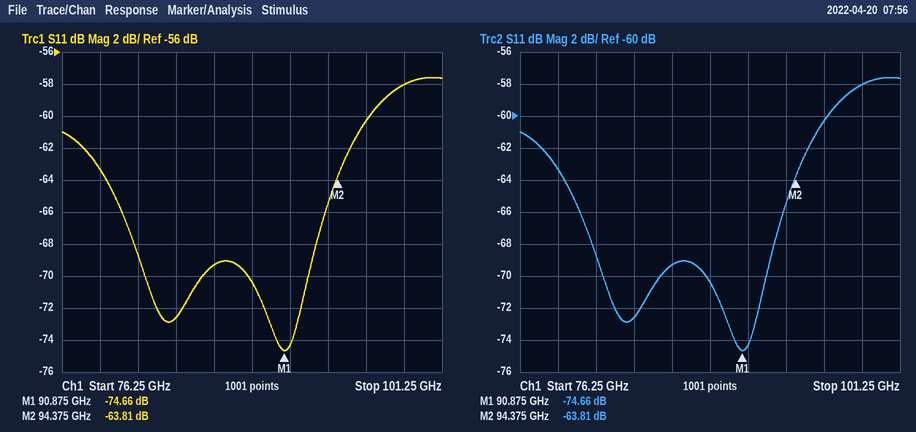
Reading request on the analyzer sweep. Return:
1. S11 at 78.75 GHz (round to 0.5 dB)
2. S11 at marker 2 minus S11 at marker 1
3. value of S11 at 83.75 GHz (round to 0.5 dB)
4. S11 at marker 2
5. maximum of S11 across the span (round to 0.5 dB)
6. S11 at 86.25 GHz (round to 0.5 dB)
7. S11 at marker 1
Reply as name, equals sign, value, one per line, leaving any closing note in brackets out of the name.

S11 at 78.75 GHz = -63.5 dB
S11 at marker 2 minus S11 at marker 1 = 10.85 dB
value of S11 at 83.75 GHz = -72.5 dB
S11 at marker 2 = -63.81 dB
maximum of S11 across the span = -57.5 dB
S11 at 86.25 GHz = -69.5 dB
S11 at marker 1 = -74.66 dB
